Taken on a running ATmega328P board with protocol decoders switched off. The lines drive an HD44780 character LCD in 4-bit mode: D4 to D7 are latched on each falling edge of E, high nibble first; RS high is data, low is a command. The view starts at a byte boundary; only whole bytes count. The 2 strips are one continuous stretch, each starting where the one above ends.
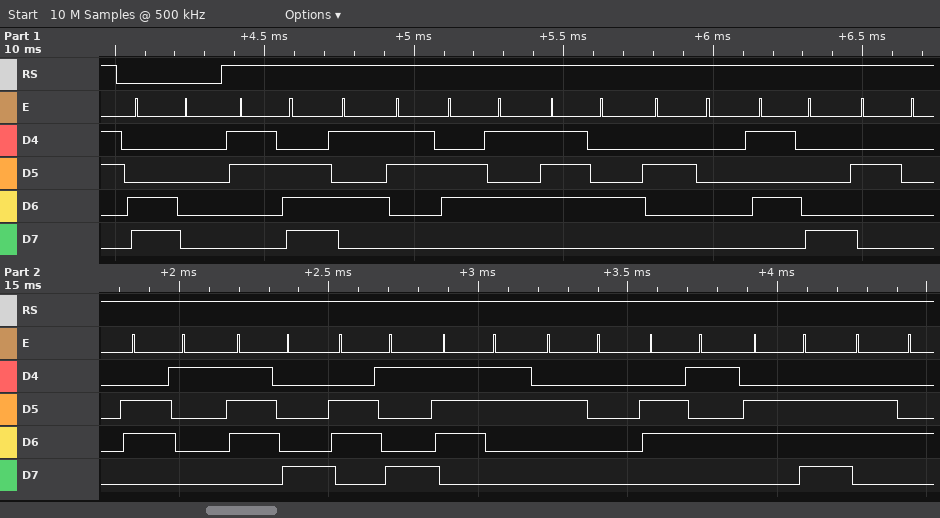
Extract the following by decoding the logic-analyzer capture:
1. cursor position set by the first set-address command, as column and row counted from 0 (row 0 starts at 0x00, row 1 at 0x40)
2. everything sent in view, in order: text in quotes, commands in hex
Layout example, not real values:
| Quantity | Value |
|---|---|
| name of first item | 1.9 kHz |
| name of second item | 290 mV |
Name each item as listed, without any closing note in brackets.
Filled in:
| Quantity | Value |
|---|---|
| cursor position set by the first set-address command, as column and row counted from 0 | column 0, row 1 |
| everything sent in view, in order: text in quotes, commands in hex | 0xC0 ">Set X axis end" |
